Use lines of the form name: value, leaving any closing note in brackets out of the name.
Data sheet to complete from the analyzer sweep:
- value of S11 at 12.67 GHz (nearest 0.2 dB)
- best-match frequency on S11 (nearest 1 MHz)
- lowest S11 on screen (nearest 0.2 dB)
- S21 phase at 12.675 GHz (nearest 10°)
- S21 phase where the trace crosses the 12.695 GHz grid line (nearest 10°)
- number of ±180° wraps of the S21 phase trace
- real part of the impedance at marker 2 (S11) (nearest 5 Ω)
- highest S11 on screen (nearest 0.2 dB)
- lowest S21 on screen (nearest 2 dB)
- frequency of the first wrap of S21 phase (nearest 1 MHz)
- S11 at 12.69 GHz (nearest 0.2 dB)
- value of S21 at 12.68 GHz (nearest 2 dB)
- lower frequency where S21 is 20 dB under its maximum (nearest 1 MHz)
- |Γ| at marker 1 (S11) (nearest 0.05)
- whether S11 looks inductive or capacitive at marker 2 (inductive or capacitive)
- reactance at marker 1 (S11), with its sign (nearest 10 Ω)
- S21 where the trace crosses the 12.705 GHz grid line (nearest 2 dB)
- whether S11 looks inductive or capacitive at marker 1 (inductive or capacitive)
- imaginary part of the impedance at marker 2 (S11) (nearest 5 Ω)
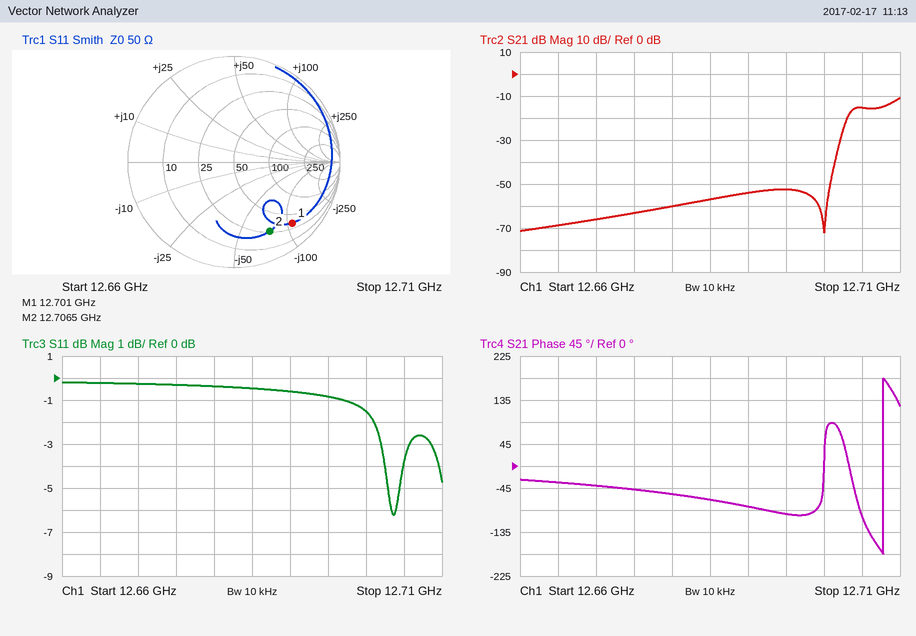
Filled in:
value of S11 at 12.67 GHz: -0.2 dB
best-match frequency on S11: 12.704 GHz
lowest S11 on screen: -6.2 dB
S21 phase at 12.675 GHz: -50°
S21 phase where the trace crosses the 12.695 GHz grid line: -100°
number of ±180° wraps of the S21 phase trace: 1
real part of the impedance at marker 2 (S11): 25 Ω
highest S11 on screen: -0.2 dB
lowest S21 on screen: -72 dB
frequency of the first wrap of S21 phase: 12.708 GHz
S11 at 12.69 GHz: -0.6 dB
value of S21 at 12.68 GHz: -60 dB
lower frequency where S21 is 20 dB under its maximum: 12.702 GHz
|Γ| at marker 1 (S11): 0.80
whether S11 looks inductive or capacitive at marker 2: capacitive
reactance at marker 1 (S11), with its sign: -110 Ω
S21 where the trace crosses the 12.705 GHz grid line: -16 dB
whether S11 looks inductive or capacitive at marker 1: capacitive
imaginary part of the impedance at marker 2 (S11): -75 Ω
